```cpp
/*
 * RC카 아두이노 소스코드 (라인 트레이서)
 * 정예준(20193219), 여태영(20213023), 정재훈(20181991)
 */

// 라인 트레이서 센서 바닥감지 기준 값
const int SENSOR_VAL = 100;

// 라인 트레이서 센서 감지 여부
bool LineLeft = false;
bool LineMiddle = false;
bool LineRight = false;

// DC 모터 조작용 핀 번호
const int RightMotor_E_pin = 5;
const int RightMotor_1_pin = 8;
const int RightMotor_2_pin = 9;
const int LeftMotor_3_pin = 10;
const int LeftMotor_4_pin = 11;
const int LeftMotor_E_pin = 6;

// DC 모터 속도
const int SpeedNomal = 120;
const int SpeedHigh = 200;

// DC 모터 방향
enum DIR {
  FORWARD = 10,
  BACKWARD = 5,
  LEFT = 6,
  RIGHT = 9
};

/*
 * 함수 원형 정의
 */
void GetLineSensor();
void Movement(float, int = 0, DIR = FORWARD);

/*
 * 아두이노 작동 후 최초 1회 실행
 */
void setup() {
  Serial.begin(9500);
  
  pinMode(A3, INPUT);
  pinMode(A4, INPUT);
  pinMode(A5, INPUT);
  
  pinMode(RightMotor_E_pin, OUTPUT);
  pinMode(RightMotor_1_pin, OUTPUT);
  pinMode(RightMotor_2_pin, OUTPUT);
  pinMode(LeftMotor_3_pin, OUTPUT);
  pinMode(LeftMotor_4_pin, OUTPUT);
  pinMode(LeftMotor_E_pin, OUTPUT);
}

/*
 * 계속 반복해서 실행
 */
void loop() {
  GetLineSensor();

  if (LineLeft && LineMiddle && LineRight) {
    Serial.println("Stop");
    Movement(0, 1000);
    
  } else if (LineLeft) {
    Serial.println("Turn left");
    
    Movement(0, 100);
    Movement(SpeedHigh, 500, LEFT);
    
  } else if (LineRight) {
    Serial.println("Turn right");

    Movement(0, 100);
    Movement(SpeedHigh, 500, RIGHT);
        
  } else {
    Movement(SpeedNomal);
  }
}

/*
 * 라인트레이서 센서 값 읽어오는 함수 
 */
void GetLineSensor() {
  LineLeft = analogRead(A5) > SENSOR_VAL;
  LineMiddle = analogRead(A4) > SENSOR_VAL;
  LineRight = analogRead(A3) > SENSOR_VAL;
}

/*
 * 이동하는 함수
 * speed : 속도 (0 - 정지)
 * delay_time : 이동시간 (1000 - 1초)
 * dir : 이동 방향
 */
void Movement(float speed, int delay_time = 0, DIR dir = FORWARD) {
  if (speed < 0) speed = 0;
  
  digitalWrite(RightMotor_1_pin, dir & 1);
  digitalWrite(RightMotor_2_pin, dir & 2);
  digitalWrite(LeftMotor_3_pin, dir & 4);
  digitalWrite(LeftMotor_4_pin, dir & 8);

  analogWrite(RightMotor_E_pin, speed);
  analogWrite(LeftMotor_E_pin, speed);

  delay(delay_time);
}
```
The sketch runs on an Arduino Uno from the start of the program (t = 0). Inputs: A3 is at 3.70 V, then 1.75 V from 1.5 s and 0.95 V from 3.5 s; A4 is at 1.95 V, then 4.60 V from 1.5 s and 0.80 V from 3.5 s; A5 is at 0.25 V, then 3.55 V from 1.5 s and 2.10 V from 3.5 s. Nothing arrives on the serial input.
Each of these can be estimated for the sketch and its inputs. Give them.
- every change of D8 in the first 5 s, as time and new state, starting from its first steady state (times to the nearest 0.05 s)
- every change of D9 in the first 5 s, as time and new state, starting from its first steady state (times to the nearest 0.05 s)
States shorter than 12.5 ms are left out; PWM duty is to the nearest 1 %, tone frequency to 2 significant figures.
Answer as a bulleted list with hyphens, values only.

- 0 s low; 0.1 s high; 0.6 s low; 0.7 s high; 1.2 s low; 1.3 s high; 1.8 s low
- 0 s high; 0.1 s low; 0.6 s high; 0.7 s low; 1.2 s high; 1.3 s low; 1.8 s high
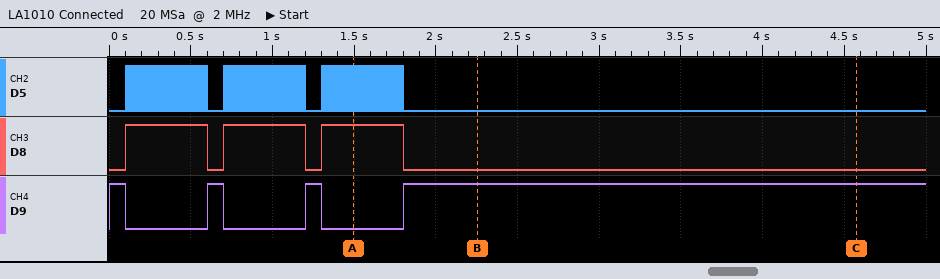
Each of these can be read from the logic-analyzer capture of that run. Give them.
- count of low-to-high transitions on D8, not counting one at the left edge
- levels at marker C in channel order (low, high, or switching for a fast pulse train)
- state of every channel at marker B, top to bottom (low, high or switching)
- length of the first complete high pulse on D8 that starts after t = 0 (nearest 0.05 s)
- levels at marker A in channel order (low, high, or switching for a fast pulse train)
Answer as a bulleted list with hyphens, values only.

- 3
- D5 low, D8 low, D9 high
- D5 low, D8 low, D9 high
- 0.50 s
- D5 switching, D8 high, D9 low
